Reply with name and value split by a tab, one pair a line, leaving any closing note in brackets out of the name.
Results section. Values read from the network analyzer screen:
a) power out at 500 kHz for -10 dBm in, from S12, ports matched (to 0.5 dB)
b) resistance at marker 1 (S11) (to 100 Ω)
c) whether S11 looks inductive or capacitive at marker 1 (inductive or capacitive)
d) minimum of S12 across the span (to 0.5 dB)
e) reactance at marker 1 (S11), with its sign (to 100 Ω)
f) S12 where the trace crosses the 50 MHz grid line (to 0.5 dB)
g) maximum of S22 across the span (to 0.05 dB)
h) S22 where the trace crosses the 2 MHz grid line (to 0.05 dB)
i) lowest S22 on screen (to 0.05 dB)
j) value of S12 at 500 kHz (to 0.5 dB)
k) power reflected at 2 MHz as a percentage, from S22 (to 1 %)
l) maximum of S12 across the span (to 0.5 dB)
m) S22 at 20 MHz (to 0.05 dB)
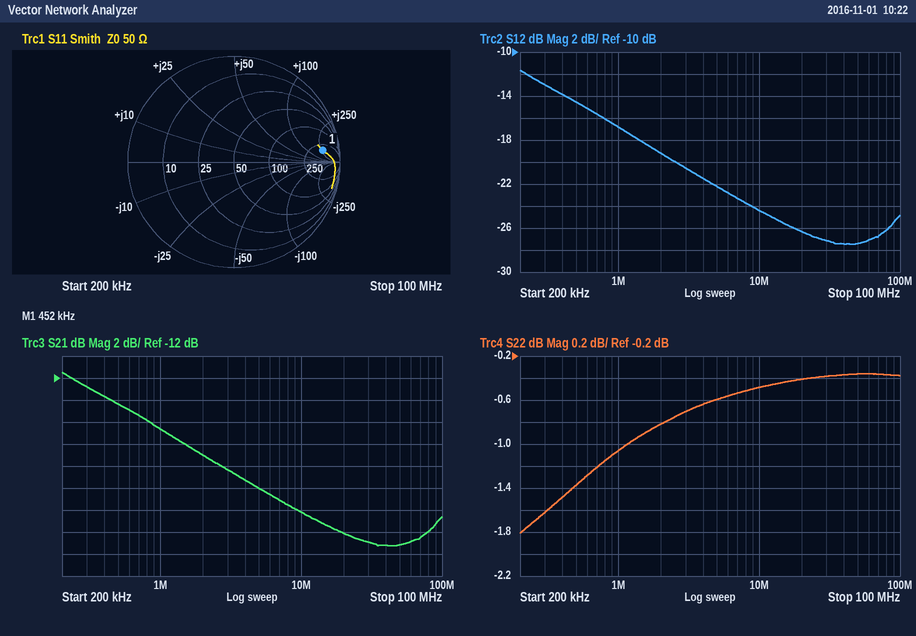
power out at 500 kHz for -10 dBm in, from S12, ports matched	-24.5 dBm
resistance at marker 1 (S11)	400 Ω
whether S11 looks inductive or capacitive at marker 1	inductive
minimum of S12 across the span	-27.5 dB
reactance at marker 1 (S11), with its sign	+300 Ω
S12 where the trace crosses the 50 MHz grid line	-27.5 dB
maximum of S22 across the span	-0.35 dB
S22 where the trace crosses the 2 MHz grid line	-0.80 dB
lowest S22 on screen	-1.80 dB
value of S12 at 500 kHz	-14.5 dB
power reflected at 2 MHz as a percentage, from S22	83 %
maximum of S12 across the span	-11.5 dB
S22 at 20 MHz	-0.40 dB
